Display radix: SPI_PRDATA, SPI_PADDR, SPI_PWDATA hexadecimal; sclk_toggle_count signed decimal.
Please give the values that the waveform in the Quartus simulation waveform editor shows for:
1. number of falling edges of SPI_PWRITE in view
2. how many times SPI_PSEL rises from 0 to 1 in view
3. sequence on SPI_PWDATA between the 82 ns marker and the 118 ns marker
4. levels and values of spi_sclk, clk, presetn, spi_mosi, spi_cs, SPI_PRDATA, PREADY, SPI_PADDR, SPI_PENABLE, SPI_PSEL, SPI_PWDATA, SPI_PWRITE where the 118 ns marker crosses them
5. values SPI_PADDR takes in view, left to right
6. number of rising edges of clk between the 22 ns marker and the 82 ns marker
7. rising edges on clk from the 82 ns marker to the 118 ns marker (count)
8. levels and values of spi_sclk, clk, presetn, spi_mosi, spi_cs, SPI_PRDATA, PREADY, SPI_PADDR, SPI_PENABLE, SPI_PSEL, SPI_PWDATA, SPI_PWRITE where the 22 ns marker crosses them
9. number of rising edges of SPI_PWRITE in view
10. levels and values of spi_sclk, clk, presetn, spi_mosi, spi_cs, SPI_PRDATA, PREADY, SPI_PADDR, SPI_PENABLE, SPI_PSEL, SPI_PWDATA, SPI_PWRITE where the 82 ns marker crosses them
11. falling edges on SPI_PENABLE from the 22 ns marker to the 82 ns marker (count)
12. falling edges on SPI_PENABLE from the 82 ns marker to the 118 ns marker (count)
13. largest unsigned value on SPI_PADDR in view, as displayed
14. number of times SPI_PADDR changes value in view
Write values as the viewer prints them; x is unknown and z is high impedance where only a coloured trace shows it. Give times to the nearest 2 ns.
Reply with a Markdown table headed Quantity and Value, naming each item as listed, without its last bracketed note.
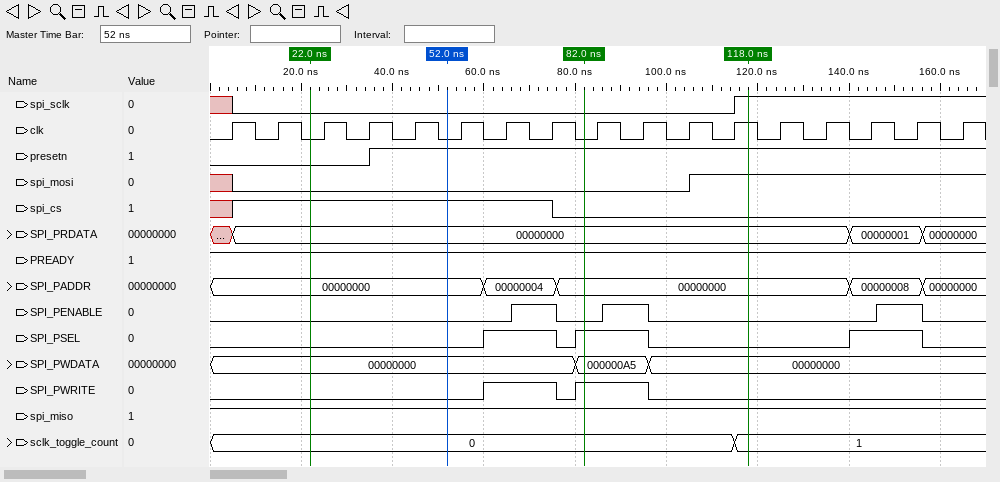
| Quantity | Value |
|---|---|
| number of falling edges of SPI_PWRITE in view | 2 |
| how many times SPI_PSEL rises from 0 to 1 in view | 3 |
| sequence on SPI_PWDATA between the 82 ns marker and the 118 ns marker | 000000A5, 00000000 |
| levels and values of spi_sclk, clk, presetn, spi_mosi, spi_cs, SPI_PRDATA, PREADY, SPI_PADDR, SPI_PENABLE, SPI_PSEL, SPI_PWDATA, SPI_PWRITE where the 118 ns marker crosses them | spi_sclk=1, clk=1, presetn=1, spi_mosi=1, spi_cs=0, SPI_PRDATA=00000000, PREADY=1, SPI_PADDR=00000000, SPI_PENABLE=0, SPI_PSEL=0, SPI_PWDATA=00000000, SPI_PWRITE=0 |
| values SPI_PADDR takes in view, left to right | 00000000, 00000004, 00000000, 00000008, 00000000 |
| number of rising edges of clk between the 22 ns marker and the 82 ns marker | 6 |
| rising edges on clk from the 82 ns marker to the 118 ns marker | 4 |
| levels and values of spi_sclk, clk, presetn, spi_mosi, spi_cs, SPI_PRDATA, PREADY, SPI_PADDR, SPI_PENABLE, SPI_PSEL, SPI_PWDATA, SPI_PWRITE where the 22 ns marker crosses them | spi_sclk=0, clk=0, presetn=0, spi_mosi=0, spi_cs=1, SPI_PRDATA=00000000, PREADY=1, SPI_PADDR=00000000, SPI_PENABLE=0, SPI_PSEL=0, SPI_PWDATA=00000000, SPI_PWRITE=0 |
| number of rising edges of SPI_PWRITE in view | 2 |
| levels and values of spi_sclk, clk, presetn, spi_mosi, spi_cs, SPI_PRDATA, PREADY, SPI_PADDR, SPI_PENABLE, SPI_PSEL, SPI_PWDATA, SPI_PWRITE where the 82 ns marker crosses them | spi_sclk=0, clk=0, presetn=1, spi_mosi=0, spi_cs=0, SPI_PRDATA=00000000, PREADY=1, SPI_PADDR=00000000, SPI_PENABLE=0, SPI_PSEL=1, SPI_PWDATA=000000A5, SPI_PWRITE=1 |
| falling edges on SPI_PENABLE from the 22 ns marker to the 82 ns marker | 1 |
| falling edges on SPI_PENABLE from the 82 ns marker to the 118 ns marker | 1 |
| largest unsigned value on SPI_PADDR in view, as displayed | 00000008 |
| number of times SPI_PADDR changes value in view | 4 |
